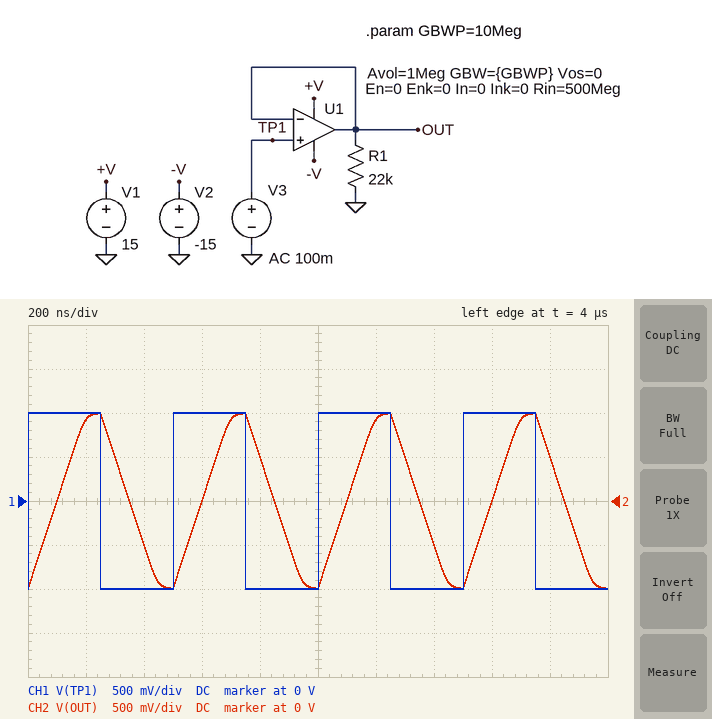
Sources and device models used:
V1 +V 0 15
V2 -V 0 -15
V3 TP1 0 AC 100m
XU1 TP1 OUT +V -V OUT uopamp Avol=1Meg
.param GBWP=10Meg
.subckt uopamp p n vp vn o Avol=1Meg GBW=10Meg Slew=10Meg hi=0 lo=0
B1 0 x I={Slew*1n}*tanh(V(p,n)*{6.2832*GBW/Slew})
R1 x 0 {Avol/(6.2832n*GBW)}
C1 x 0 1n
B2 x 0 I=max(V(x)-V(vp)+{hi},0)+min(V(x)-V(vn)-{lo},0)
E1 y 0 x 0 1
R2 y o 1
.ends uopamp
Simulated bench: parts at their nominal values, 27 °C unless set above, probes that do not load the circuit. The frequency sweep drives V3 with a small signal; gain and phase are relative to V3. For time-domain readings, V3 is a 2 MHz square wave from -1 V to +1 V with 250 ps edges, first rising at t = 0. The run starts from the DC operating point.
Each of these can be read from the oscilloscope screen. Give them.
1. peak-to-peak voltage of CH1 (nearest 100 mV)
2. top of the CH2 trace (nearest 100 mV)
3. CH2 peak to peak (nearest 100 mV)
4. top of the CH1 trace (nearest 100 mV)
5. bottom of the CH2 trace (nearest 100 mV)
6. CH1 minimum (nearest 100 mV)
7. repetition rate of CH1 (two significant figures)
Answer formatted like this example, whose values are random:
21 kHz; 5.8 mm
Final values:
2.0 V; 1.0 V; 2.0 V; 1.0 V; -1.0 V; -1.0 V; 2.0 MHz
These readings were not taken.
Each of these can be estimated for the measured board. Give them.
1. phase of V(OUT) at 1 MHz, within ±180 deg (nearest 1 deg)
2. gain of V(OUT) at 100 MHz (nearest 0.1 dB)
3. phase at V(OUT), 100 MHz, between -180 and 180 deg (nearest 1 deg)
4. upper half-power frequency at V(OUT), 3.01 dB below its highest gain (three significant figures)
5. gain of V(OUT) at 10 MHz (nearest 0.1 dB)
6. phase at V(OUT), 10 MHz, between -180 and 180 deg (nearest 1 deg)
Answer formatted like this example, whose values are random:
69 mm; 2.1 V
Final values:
-6 deg; -20.0 dB; -84 deg; 10.0 MHz; -3.0 dB; -45 deg
